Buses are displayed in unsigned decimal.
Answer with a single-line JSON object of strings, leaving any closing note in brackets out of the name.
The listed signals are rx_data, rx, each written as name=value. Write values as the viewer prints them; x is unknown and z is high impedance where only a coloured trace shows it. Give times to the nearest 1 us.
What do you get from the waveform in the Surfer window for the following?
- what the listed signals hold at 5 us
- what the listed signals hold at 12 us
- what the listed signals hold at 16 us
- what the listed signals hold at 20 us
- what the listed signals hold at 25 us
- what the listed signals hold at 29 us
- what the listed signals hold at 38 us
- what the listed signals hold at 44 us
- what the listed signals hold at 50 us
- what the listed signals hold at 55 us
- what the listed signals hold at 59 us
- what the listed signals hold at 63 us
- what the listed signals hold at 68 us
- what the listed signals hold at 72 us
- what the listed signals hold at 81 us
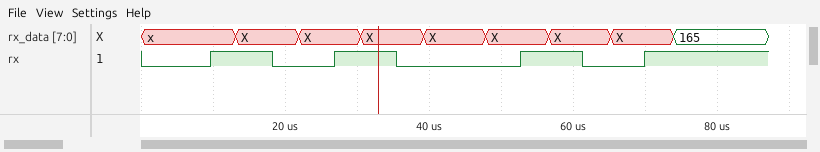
{"what the listed signals hold at 5 us": "rx_data=x, rx=0", "what the listed signals hold at 12 us": "rx_data=x, rx=1", "what the listed signals hold at 16 us": "rx_data=X, rx=1", "what the listed signals hold at 20 us": "rx_data=X, rx=0", "what the listed signals hold at 25 us": "rx_data=X, rx=0", "what the listed signals hold at 29 us": "rx_data=X, rx=1", "what the listed signals hold at 38 us": "rx_data=X, rx=0", "what the listed signals hold at 44 us": "rx_data=X, rx=0", "what the listed signals hold at 50 us": "rx_data=X, rx=0", "what the listed signals hold at 55 us": "rx_data=X, rx=1", "what the listed signals hold at 59 us": "rx_data=X, rx=1", "what the listed signals hold at 63 us": "rx_data=X, rx=0", "what the listed signals hold at 68 us": "rx_data=X, rx=0", "what the listed signals hold at 72 us": "rx_data=X, rx=1", "what the listed signals hold at 81 us": "rx_data=165, rx=1"}
